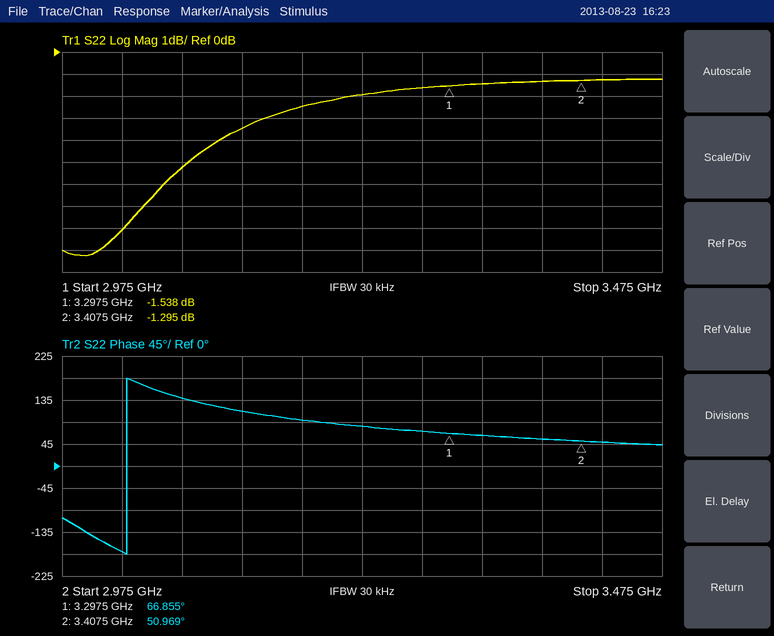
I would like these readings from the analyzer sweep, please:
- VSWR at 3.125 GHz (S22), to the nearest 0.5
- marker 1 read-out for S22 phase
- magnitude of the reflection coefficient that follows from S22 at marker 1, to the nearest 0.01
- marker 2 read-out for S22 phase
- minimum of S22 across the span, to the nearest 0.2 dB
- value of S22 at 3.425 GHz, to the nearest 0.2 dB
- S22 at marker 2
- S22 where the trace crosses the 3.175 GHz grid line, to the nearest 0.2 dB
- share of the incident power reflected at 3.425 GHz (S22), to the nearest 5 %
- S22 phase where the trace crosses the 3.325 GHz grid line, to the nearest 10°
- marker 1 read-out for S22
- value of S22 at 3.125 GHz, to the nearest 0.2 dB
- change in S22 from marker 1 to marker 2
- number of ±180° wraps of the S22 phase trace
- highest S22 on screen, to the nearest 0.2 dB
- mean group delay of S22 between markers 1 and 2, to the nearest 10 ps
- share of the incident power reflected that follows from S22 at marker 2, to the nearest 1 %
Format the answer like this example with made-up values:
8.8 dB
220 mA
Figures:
5.0
66.855°
0.84
50.969°
-9.2 dB
-1.2 dB
-1.295 dB
-2.4 dB
75 %
60°
-1.538 dB
-3.4 dB
0.243 dB
1
-1.2 dB
400 ps
74 %
